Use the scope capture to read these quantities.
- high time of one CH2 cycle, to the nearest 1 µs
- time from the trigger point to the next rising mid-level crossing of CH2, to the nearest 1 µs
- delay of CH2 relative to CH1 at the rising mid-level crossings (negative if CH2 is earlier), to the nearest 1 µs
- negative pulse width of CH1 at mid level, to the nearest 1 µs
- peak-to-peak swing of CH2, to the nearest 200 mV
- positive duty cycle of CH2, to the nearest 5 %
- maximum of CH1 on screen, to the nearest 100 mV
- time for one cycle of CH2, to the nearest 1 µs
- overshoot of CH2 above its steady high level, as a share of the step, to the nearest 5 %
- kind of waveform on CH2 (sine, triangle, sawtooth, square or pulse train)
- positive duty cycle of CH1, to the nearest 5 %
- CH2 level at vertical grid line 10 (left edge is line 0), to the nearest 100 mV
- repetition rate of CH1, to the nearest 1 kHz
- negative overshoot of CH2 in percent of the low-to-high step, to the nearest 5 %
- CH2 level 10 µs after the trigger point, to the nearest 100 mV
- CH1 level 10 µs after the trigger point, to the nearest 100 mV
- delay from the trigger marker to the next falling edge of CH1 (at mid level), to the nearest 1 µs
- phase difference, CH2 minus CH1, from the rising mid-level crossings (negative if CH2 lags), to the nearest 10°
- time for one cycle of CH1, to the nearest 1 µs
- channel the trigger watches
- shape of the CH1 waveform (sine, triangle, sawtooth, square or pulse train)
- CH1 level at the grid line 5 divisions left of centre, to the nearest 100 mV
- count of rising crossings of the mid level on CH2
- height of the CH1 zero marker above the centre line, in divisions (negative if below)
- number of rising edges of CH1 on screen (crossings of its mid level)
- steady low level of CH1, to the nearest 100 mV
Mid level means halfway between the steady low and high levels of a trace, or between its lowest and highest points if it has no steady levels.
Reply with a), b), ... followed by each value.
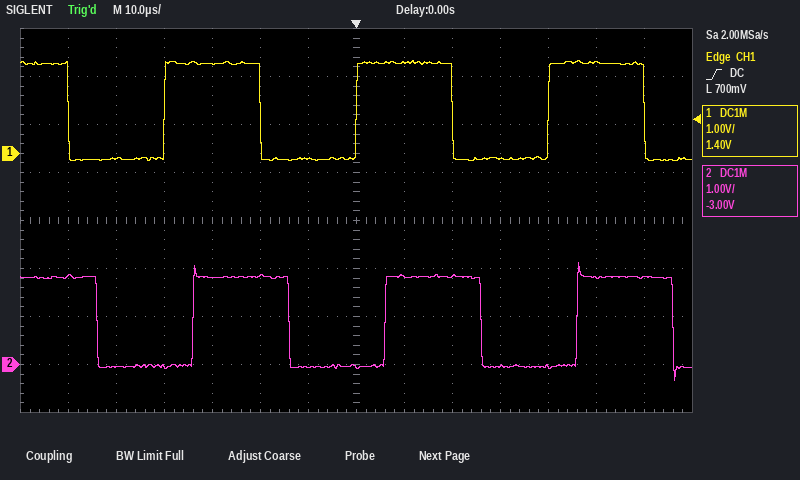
a) 20 µs
b) 6 µs
c) +6 µs
d) 20 µs
e) 2.4 V
f) 50 %
g) 1.9 V
h) 40 µs
i) 15 %
j) square
k) 50 %
l) 0.0 V
m) 25 kHz
n) 15 %
o) 1.8 V
p) 1.9 V
q) 20 µs
r) -50°
s) 40 µs
t) CH1
u) square
v) -100 mV
w) 3
x) +1.4 div
y) 3
z) -100 mV
